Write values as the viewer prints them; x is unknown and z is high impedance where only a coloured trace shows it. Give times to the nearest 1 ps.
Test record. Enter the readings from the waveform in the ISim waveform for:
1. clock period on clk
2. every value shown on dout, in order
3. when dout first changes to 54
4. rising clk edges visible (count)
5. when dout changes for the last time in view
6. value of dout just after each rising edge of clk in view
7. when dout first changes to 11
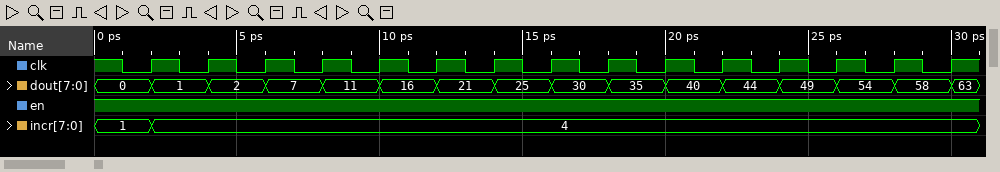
2 ps
0, 1, 2, 7, 11, 16, 21, 25, 30, 35, 40, 44, 49, 54, 58, 63
26 ps
15
30 ps
1, 2, 7, 11, 16, 21, 25, 30, 35, 40, 44, 49, 54, 58, 63
8 ps
